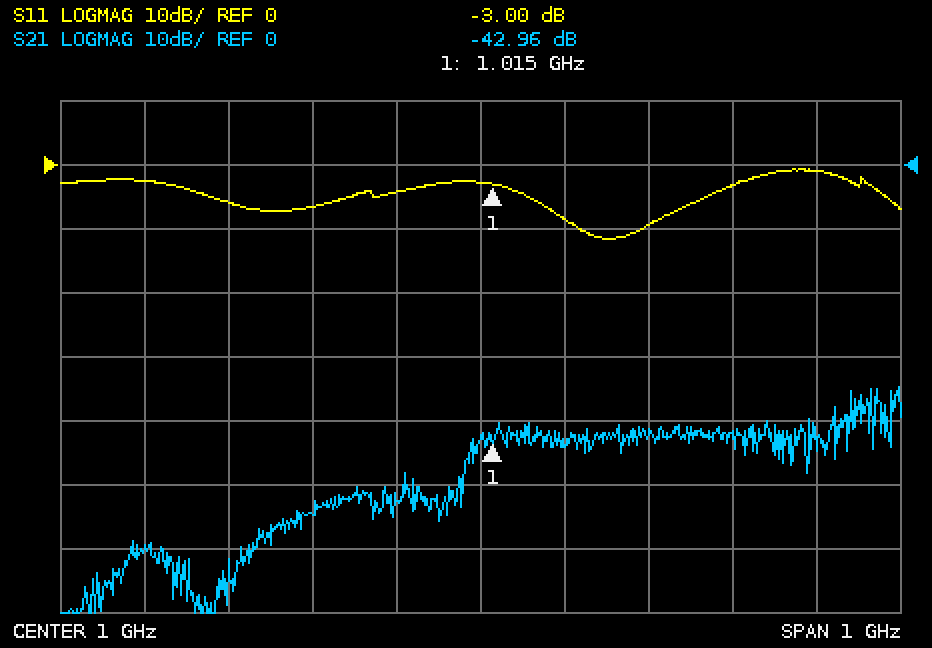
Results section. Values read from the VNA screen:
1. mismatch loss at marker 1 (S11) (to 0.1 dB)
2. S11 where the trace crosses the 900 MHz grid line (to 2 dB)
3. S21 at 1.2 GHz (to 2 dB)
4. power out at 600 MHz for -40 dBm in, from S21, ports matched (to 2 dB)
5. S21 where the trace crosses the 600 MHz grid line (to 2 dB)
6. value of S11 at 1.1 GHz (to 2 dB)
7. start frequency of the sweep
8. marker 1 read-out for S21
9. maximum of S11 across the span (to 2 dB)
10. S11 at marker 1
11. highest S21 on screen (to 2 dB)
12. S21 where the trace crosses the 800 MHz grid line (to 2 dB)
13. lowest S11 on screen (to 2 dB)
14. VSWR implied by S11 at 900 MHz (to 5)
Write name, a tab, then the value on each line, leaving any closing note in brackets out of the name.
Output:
mismatch loss at marker 1 (S11)	3.0 dB
S11 where the trace crosses the 900 MHz grid line	-4 dB
S21 at 1.2 GHz	-42 dB
power out at 600 MHz for -40 dBm in, from S21, ports matched	-100 dBm
S21 where the trace crosses the 600 MHz grid line	-60 dB
value of S11 at 1.1 GHz	-8 dB
start frequency of the sweep	500 MHz
marker 1 read-out for S21	-42.96 dB
maximum of S11 across the span	0 dB
S11 at marker 1	-3.00 dB
highest S21 on screen	-34 dB
S21 where the trace crosses the 800 MHz grid line	-54 dB
lowest S11 on screen	-12 dB
VSWR implied by S11 at 900 MHz	5
